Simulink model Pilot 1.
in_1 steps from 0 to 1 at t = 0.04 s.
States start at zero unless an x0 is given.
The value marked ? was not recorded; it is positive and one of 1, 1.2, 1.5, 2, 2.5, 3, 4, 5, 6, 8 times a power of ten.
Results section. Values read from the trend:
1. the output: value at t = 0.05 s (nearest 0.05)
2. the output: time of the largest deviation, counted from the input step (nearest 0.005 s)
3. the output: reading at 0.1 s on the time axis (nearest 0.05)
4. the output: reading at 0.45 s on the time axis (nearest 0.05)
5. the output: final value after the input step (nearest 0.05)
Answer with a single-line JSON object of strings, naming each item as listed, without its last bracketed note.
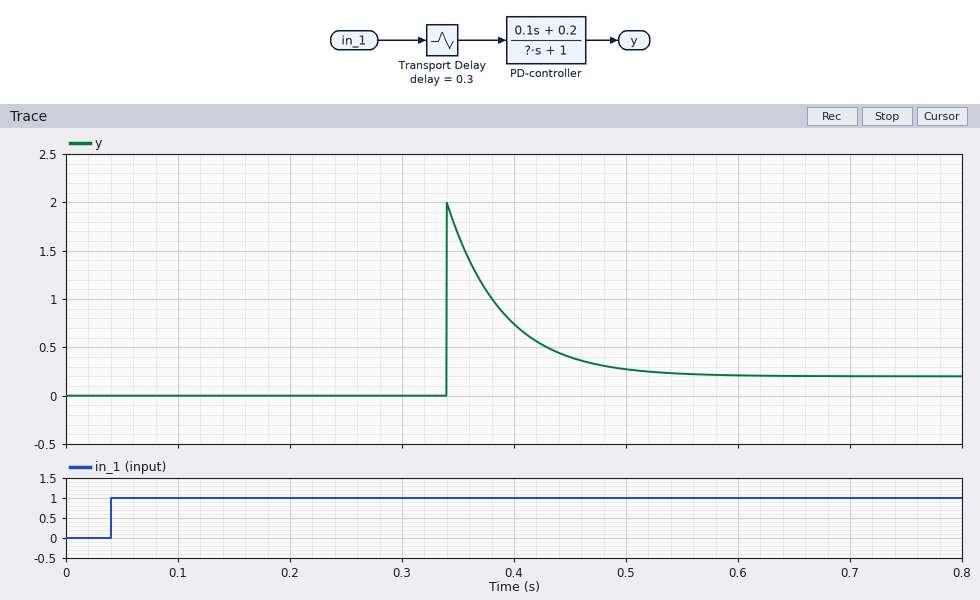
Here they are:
{"the output: value at t = 0.05 s": "0.00", "the output: time of the largest deviation, counted from the input step": "0.300 s", "the output: reading at 0.1 s on the time axis": "0.00", "the output: reading at 0.45 s on the time axis": "0.40", "the output: final value after the input step": "0.20"}
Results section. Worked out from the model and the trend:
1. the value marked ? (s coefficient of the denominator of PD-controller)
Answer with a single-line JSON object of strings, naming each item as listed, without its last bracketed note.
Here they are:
{"the value marked ?": "0.05"}
